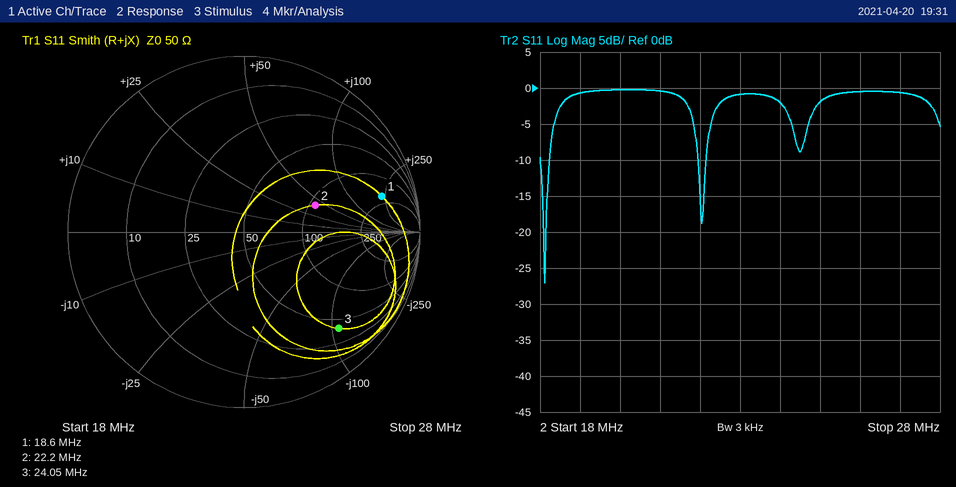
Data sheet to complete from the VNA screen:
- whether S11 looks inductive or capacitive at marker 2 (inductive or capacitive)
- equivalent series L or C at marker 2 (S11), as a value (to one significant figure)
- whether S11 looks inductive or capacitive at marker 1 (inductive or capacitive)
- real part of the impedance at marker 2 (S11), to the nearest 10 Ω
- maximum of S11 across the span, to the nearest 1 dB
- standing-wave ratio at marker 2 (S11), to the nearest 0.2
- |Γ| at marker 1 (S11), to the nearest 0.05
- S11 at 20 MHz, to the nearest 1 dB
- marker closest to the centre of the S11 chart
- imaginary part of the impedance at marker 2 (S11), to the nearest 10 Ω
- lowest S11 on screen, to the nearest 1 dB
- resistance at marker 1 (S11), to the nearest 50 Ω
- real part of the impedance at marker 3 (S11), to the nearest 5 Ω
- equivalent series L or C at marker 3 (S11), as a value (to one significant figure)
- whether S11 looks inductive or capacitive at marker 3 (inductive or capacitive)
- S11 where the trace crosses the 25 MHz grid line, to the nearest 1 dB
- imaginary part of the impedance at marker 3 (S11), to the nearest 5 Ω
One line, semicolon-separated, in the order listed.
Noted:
inductive; 300 nH; inductive; 110 Ω; 0 dB; 2.6; 0.80; 0 dB; marker 2; +40 Ω; -27 dB; 200 Ω; 40 Ω; 60 pF; capacitive; -2 dB; -105 Ω
